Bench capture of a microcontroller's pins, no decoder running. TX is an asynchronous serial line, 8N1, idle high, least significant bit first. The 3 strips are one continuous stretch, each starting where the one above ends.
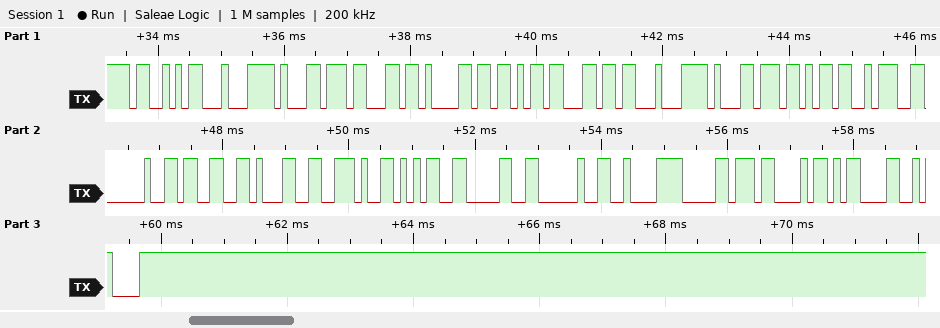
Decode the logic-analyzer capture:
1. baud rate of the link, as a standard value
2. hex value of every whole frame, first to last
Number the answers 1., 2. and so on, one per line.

1. 9600 baud
2. 53 C4 B1 63 61 6B 6C C4 B1 6B 3A 20 33 31 2E 35 30 20 C2 B0 43 0D 0A
